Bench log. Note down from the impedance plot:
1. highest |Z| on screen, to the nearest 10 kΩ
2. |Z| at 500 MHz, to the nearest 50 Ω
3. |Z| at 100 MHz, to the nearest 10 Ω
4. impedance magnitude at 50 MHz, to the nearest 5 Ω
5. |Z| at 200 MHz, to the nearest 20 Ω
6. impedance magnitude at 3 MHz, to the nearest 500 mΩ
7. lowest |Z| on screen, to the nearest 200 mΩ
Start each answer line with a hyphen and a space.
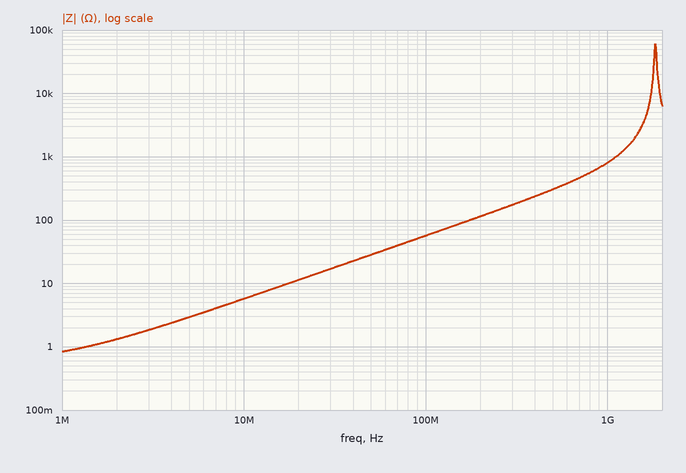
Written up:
- 60 kΩ
- 300 Ω
- 60 Ω
- 30 Ω
- 120 Ω
- 2.0 Ω
- 800 mΩ
